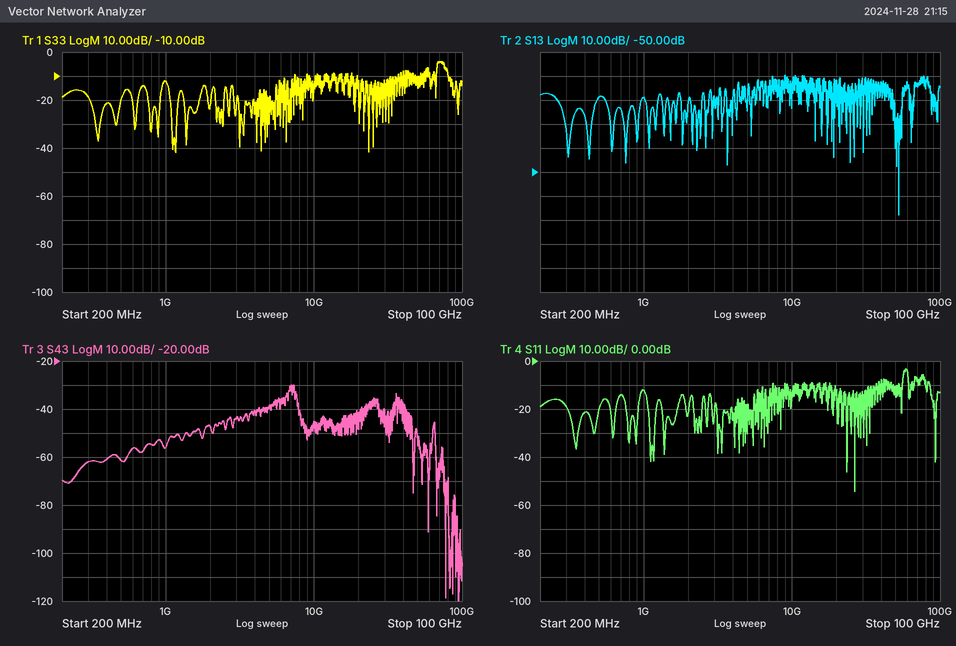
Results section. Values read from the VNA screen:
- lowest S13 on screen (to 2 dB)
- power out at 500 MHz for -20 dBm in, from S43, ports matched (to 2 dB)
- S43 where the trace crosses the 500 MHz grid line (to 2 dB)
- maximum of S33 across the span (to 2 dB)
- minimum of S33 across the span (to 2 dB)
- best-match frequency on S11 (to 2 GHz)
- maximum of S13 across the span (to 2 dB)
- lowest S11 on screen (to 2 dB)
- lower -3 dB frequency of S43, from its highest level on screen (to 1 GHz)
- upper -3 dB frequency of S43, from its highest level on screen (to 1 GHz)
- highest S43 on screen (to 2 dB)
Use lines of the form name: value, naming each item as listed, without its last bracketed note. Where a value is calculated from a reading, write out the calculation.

lowest S13 on screen: -68 dB
power out at 500 MHz for -20 dBm in, from S43, ports matched: -20 dBm + (-62 dB) = -82 dBm
S43 where the trace crosses the 500 MHz grid line: -62 dB
maximum of S33 across the span: -4 dB
minimum of S33 across the span: -42 dB
best-match frequency on S11: 26 GHz
maximum of S13 across the span: -10 dB
lowest S11 on screen: -54 dB
lower -3 dB frequency of S43, from its highest level on screen: 7 GHz
upper -3 dB frequency of S43, from its highest level on screen: 7 GHz
highest S43 on screen: -30 dB
